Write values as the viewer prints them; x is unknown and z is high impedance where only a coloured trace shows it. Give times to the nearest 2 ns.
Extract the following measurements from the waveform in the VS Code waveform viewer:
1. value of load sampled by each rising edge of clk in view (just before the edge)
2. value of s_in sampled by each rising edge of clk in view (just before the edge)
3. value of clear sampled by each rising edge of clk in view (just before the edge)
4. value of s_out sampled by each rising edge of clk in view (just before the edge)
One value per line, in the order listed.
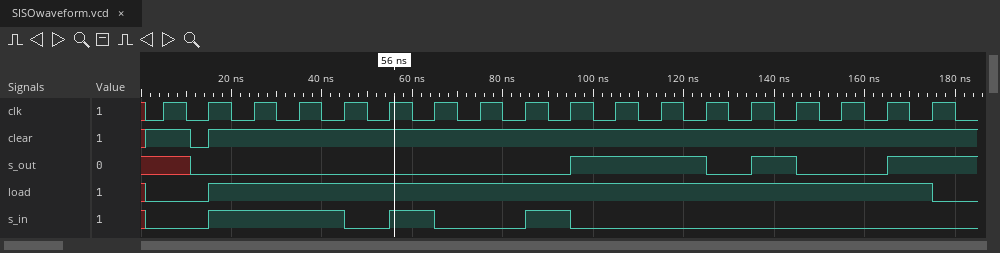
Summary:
0 0 1 1 1 1 1 1 1 1 1 1 1 1 1 1 1 1
0 0 1 1 1 0 1 0 0 1 0 0 0 0 0 0 0 0
1 0 1 1 1 1 1 1 1 1 1 1 1 1 1 1 1 1
x 0 0 0 0 0 0 0 0 0 1 1 1 0 1 0 0 1
